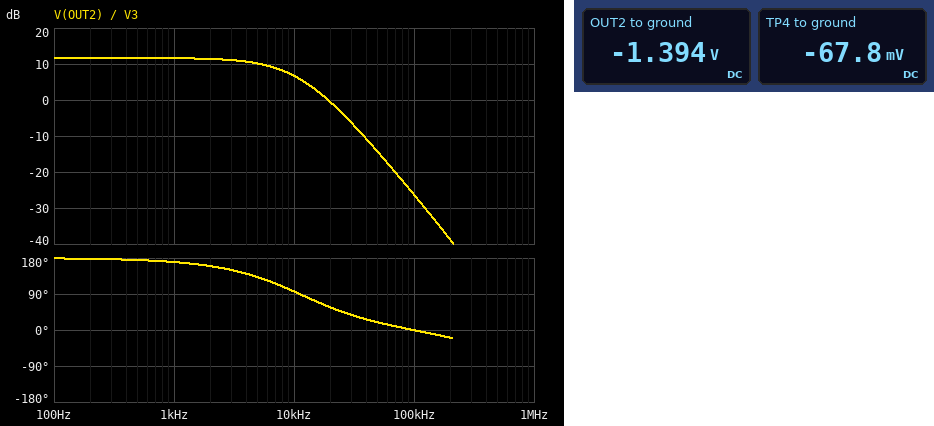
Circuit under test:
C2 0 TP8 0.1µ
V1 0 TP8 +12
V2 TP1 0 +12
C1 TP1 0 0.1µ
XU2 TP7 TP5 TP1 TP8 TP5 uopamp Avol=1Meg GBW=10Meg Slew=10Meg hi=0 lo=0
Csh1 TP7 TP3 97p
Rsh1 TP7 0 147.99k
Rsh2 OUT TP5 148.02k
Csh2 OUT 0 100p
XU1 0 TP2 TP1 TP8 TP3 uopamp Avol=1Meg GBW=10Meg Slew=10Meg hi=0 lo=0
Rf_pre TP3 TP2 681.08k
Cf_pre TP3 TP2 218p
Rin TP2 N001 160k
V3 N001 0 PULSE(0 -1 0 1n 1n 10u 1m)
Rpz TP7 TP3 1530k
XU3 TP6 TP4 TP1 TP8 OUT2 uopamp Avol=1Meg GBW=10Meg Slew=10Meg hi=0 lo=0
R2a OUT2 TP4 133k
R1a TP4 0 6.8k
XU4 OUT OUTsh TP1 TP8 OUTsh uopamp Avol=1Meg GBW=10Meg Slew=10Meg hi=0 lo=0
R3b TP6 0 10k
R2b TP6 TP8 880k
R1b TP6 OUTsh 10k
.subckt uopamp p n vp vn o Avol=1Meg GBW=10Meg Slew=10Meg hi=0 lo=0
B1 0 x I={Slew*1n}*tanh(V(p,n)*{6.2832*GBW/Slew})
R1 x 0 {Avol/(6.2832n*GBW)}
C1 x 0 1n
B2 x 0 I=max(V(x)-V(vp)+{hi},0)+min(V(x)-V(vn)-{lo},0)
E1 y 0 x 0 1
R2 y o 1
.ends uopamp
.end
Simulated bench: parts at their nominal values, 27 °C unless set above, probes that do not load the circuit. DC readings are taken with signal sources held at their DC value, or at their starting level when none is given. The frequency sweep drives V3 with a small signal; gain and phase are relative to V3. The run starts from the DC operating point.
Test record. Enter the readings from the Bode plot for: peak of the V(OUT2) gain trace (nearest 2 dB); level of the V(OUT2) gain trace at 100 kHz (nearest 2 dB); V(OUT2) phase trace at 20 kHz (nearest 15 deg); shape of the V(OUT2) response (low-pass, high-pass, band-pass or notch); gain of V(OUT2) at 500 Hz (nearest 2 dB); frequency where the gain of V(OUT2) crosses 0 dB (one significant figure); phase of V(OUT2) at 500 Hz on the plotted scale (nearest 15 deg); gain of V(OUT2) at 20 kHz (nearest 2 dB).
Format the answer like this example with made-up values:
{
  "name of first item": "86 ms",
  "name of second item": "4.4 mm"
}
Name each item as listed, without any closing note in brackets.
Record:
{
  "peak of the V(OUT2) gain trace": "12 dB",
  "level of the V(OUT2) gain trace at 100 kHz": "-26 dB",
  "V(OUT2) phase trace at 20 kHz": "60 deg",
  "shape of the V(OUT2) response": "low-pass",
  "gain of V(OUT2) at 500 Hz": "12 dB",
  "frequency where the gain of V(OUT2) crosses 0 dB": "20 kHz",
  "phase of V(OUT2) at 500 Hz on the plotted scale": "180 deg",
  "gain of V(OUT2) at 20 kHz": "0 dB"
}
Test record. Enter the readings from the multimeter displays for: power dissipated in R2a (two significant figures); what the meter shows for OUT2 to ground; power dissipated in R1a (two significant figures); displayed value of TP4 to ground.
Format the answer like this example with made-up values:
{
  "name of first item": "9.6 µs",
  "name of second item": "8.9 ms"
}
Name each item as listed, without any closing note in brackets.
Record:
{
  "power dissipated in R2a": "13 µW",
  "what the meter shows for OUT2 to ground": "-1.394 V",
  "power dissipated in R1a": "680 nW",
  "displayed value of TP4 to ground": "-67.8 mV"
}
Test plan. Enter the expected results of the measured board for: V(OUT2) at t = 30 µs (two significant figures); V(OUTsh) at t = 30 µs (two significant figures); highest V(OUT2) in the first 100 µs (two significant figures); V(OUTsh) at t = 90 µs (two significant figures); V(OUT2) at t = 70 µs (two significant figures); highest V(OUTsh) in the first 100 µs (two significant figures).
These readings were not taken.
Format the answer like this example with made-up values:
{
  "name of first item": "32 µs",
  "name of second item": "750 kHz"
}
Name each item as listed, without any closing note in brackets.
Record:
{
  "V(OUT2) at t = 30 µs": "-570 mV",
  "V(OUTsh) at t = 30 µs": "80 mV",
  "highest V(OUT2) in the first 100 µs": "-400 mV",
  "V(OUTsh) at t = 90 µs": "3.8 mV",
  "V(OUT2) at t = 70 µs": "-1.3 V",
  "highest V(OUTsh) in the first 100 µs": "97 mV"
}
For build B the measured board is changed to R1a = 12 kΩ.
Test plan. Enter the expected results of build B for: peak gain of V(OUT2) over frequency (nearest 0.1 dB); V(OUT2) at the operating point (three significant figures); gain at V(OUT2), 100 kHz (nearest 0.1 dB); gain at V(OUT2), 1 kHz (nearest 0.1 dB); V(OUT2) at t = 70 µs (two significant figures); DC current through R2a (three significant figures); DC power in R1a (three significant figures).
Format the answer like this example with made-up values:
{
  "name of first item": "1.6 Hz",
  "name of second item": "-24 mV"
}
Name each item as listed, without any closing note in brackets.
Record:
{
  "peak gain of V(OUT2) over frequency": "7.1 dB",
  "V(OUT2) at the operating point": "-819 mV",
  "gain at V(OUT2), 100 kHz": "-30.8 dB",
  "gain at V(OUT2), 1 kHz": "7.0 dB",
  "V(OUT2) at t = 70 µs": "-750 mV",
  "DC current through R2a": "5.65 µA",
  "DC power in R1a": "383 nW"
}
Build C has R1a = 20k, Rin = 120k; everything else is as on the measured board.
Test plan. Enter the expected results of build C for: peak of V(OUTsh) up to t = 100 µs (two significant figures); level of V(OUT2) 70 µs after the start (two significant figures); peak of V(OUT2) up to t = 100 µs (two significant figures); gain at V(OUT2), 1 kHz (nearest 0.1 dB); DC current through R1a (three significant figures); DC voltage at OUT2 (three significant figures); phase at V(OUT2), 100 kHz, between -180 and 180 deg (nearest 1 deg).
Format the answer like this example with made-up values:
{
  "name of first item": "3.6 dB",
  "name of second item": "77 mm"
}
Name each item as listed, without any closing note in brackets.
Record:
{
  "peak of V(OUTsh) up to t = 100 µs": "130 mV",
  "level of V(OUT2) 70 µs after the start": "-460 mV",
  "peak of V(OUT2) up to t = 100 µs": "-27 mV",
  "gain at V(OUT2), 1 kHz": "5.5 dB",
  "DC current through R1a": "3.39 µA",
  "DC voltage at OUT2": "-519 mV",
  "phase at V(OUT2), 100 kHz, between -180 and 180 deg": "7 deg"
}
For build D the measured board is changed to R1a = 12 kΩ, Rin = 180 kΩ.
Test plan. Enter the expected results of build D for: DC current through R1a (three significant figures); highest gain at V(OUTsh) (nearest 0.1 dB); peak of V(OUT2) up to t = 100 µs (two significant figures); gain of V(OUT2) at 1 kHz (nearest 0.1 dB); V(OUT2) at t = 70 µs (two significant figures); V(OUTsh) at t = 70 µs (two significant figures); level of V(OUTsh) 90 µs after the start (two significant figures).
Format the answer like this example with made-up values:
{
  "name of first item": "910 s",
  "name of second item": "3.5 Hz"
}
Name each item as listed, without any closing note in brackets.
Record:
{
  "DC current through R1a": "5.65 µA",
  "highest gain at V(OUTsh)": "-9.5 dB",
  "peak of V(OUT2) up to t = 100 µs": "-300 mV",
  "gain of V(OUT2) at 1 kHz": "6.0 dB",
  "V(OUT2) at t = 70 µs": "-750 mV",
  "V(OUTsh) at t = 70 µs": "11 mV",
  "level of V(OUTsh) 90 µs after the start": "3.4 mV"
}
